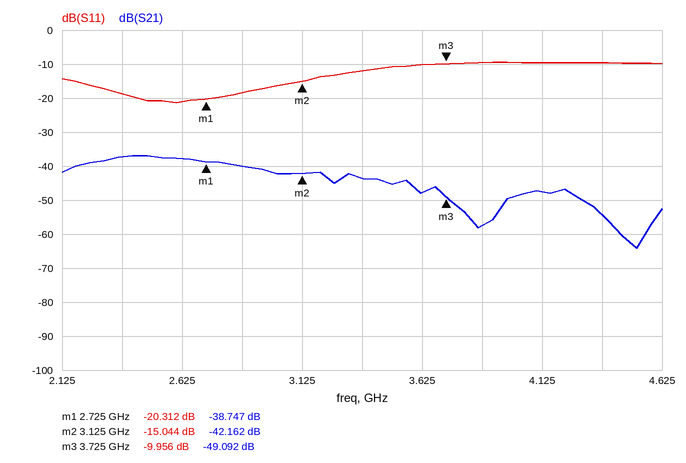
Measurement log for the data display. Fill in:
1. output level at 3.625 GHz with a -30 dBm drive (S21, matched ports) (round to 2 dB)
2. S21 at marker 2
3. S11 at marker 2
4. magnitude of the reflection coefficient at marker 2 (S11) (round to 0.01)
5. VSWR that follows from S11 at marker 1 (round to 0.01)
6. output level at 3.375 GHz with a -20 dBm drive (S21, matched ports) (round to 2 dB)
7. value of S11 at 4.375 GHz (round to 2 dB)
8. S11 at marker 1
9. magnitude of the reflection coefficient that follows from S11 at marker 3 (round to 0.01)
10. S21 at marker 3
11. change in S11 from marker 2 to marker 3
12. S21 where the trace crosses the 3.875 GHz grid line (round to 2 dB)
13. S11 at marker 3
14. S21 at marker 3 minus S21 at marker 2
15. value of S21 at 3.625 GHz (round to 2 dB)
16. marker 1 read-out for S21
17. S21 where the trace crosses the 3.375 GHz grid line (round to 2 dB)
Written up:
-78 dBm
-42.162 dB
-15.044 dB
0.18
1.21
-64 dBm
-10 dB
-20.312 dB
0.32
-49.092 dB
5.088 dB
-58 dB
-9.956 dB
-6.930 dB
-48 dB
-38.747 dB
-44 dB
